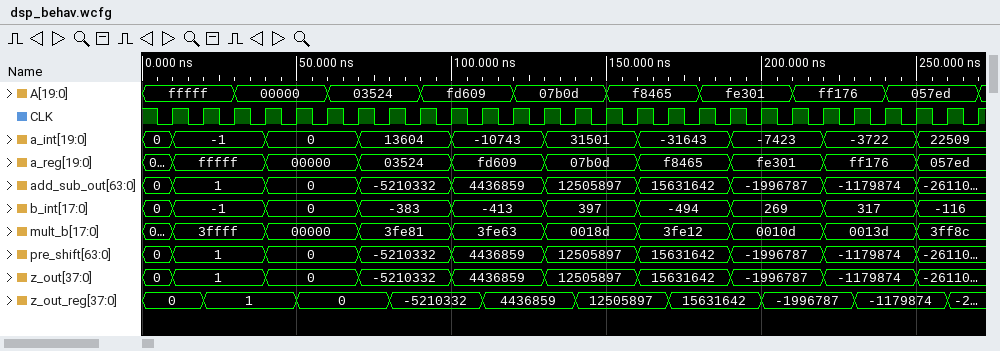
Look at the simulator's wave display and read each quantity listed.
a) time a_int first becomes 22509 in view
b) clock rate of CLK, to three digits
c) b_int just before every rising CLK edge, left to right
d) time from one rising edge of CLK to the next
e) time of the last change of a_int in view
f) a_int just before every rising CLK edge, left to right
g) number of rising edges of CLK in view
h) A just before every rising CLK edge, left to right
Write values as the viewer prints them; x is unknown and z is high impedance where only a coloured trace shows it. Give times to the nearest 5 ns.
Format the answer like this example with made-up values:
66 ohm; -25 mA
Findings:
250 ns; 100 MHz; 0, -1, -1, -1, 0, 0, 0, -383, -383, -383, -413, -413, -413, 397, 397, 397, -494, -494, -494, 269, 269, 269, 317, 317, 317, -116, -116; 10 ns; 250 ns; 0, -1, -1, -1, 0, 0, 0, 13604, 13604, 13604, -10743, -10743, -10743, 31501, 31501, 31501, -31643, -31643, -31643, -7423, -7423, -7423, -3722, -3722, -3722, 22509, 22509; 27; fffff, fffff, fffff, 00000, 00000, 00000, 03524, 03524, 03524, fd609, fd609, fd609, 07b0d, 07b0d, 07b0d, f8465, f8465, f8465, fe301, fe301, fe301, ff176, ff176, ff176, 057ed, 057ed, 057ed
